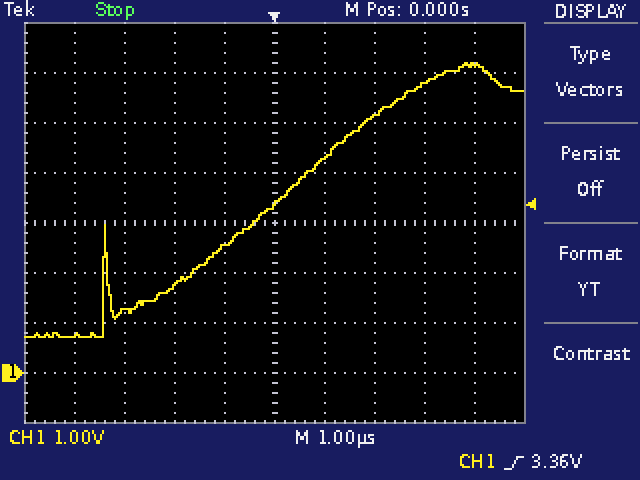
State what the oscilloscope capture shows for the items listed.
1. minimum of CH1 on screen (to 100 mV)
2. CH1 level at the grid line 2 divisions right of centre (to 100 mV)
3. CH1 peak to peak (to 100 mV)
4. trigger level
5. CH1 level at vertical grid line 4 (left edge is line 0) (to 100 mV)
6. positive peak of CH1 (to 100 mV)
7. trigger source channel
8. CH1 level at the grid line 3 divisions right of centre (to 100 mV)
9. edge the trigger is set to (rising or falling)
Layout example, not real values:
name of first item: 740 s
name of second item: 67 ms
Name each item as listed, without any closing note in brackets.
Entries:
minimum of CH1 on screen: 700 mV
CH1 level at the grid line 2 divisions right of centre: 5.1 V
CH1 peak to peak: 5.5 V
trigger level: 3.36 V
CH1 level at vertical grid line 4 (left edge is line 0): 2.5 V
positive peak of CH1: 6.2 V
trigger source channel: CH1
CH1 level at the grid line 3 divisions right of centre: 5.8 V
edge the trigger is set to: rising
